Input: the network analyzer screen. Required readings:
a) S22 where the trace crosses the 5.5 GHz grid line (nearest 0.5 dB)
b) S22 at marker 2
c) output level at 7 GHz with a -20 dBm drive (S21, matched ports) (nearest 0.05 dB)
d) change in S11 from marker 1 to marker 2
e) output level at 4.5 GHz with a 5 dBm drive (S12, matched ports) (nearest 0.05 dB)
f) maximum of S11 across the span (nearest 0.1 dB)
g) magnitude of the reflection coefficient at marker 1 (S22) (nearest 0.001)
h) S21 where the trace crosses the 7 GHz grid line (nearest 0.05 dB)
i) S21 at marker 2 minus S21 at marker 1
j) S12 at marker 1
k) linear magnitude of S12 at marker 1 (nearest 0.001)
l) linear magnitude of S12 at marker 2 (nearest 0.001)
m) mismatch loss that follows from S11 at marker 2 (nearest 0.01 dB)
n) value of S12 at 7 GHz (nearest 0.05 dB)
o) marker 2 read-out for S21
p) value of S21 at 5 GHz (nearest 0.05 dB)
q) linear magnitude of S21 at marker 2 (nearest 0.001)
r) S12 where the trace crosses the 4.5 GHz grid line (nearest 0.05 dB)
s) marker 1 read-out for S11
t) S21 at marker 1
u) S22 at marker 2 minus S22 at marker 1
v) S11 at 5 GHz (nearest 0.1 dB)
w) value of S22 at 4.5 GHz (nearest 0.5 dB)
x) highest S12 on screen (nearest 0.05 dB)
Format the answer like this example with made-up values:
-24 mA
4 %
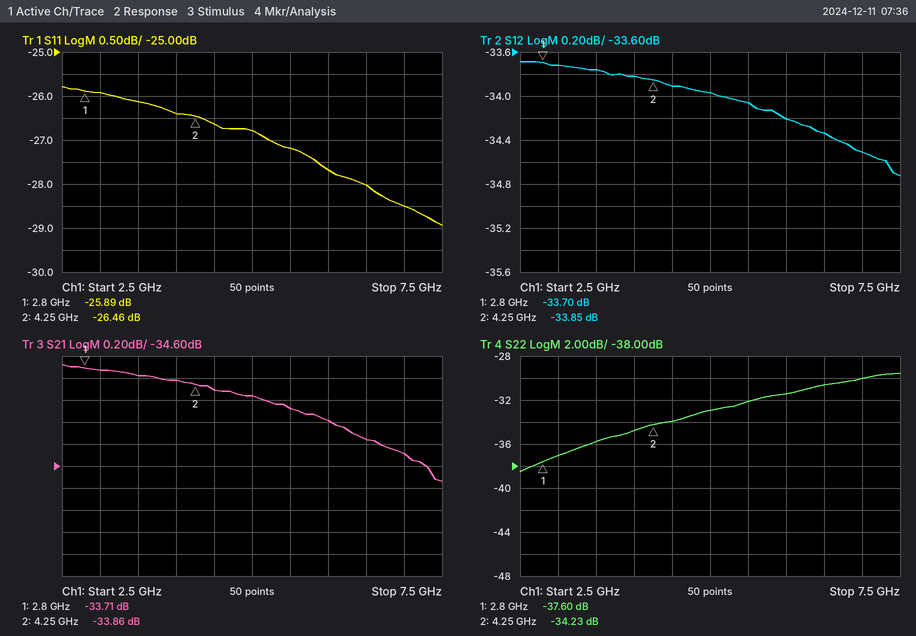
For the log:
-32.0 dB
-34.23 dB
-54.50 dBm
-0.57 dB
-28.90 dBm
-25.8 dB
0.013
-34.50 dB
-0.15 dB
-33.70 dB
0.021
0.020
0.01 dB
-34.50 dB
-33.86 dB
-33.95 dB
0.020
-33.90 dB
-25.89 dB
-33.71 dB
3.37 dB
-26.8 dB
-34.0 dB
-33.70 dB
